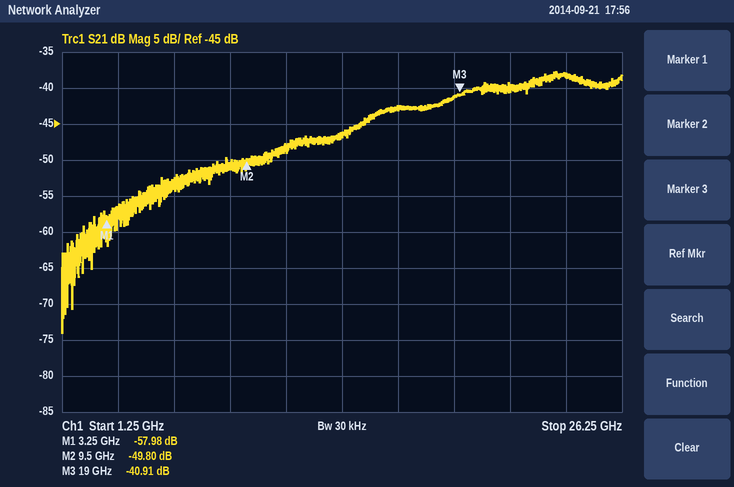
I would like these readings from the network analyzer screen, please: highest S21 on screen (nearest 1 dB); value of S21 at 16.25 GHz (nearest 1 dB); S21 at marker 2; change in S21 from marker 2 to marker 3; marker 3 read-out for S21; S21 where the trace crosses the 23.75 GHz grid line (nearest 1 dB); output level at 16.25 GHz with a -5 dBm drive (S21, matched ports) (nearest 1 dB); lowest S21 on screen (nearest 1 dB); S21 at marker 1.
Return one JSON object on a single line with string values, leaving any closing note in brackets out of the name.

{"highest S21 on screen": "-38 dB", "value of S21 at 16.25 GHz": "-43 dB", "S21 at marker 2": "-49.80 dB", "change in S21 from marker 2 to marker 3": "8.89 dB", "marker 3 read-out for S21": "-40.91 dB", "S21 where the trace crosses the 23.75 GHz grid line": "-38 dB", "output level at 16.25 GHz with a -5 dBm drive (S21, matched ports)": "-48 dBm", "lowest S21 on screen": "-74 dB", "S21 at marker 1": "-57.98 dB"}
